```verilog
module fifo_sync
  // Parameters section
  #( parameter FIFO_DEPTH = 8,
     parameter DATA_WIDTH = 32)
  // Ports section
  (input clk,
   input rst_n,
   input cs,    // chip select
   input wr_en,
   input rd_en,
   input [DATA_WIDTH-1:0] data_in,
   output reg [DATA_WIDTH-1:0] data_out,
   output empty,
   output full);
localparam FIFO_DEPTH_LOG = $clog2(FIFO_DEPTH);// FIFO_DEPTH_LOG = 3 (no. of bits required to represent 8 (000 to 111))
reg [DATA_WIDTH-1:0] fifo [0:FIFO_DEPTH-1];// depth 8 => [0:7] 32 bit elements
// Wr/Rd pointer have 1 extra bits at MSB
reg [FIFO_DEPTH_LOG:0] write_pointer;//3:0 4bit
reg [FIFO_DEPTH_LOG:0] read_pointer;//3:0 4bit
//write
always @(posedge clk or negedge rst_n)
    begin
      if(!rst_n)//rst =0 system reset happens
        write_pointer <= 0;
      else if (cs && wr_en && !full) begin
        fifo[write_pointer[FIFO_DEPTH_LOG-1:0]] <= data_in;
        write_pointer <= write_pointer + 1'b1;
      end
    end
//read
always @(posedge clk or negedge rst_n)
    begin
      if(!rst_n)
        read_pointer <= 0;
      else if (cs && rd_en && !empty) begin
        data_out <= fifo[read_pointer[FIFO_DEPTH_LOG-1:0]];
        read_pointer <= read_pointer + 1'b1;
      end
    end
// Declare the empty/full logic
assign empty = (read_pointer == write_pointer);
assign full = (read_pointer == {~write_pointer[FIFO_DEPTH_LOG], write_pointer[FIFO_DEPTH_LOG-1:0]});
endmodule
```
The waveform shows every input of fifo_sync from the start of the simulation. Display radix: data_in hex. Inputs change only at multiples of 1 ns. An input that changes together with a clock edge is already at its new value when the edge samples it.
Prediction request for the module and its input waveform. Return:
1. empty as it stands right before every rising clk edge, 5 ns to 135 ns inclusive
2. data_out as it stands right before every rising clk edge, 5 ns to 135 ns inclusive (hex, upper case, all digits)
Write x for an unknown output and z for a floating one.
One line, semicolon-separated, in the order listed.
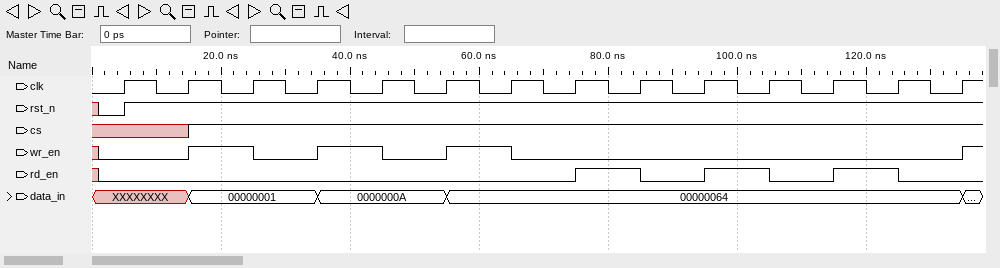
1 1 0 0 0 0 0 0 0 0 0 0 1 1; x, x, x, x, x, x, x, x, 00000001, 00000001, 0000000A, 0000000A, 00000064, 00000064
